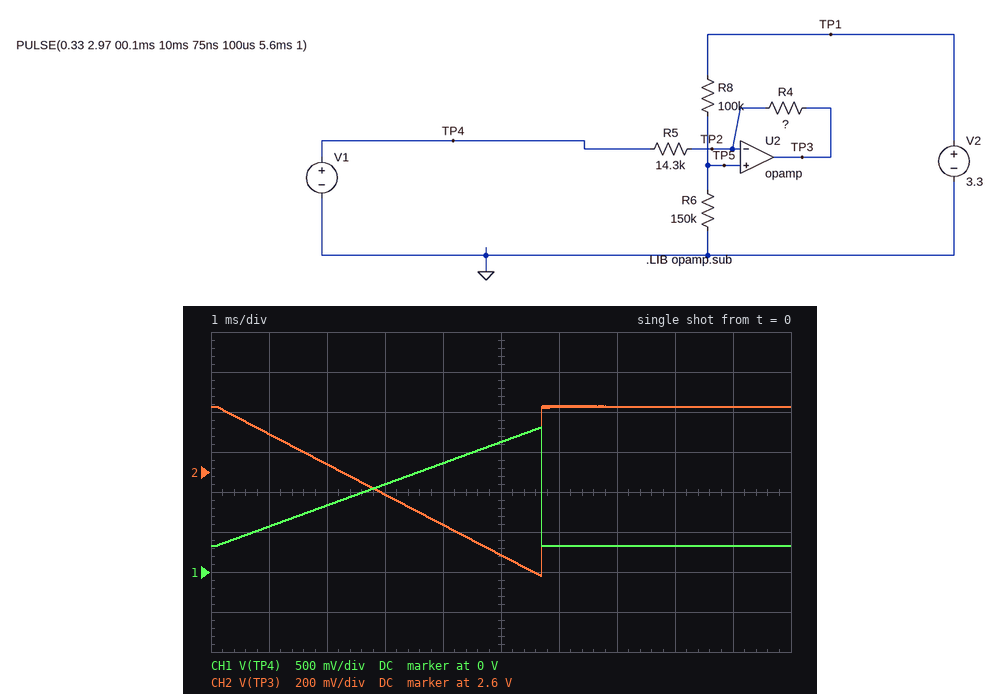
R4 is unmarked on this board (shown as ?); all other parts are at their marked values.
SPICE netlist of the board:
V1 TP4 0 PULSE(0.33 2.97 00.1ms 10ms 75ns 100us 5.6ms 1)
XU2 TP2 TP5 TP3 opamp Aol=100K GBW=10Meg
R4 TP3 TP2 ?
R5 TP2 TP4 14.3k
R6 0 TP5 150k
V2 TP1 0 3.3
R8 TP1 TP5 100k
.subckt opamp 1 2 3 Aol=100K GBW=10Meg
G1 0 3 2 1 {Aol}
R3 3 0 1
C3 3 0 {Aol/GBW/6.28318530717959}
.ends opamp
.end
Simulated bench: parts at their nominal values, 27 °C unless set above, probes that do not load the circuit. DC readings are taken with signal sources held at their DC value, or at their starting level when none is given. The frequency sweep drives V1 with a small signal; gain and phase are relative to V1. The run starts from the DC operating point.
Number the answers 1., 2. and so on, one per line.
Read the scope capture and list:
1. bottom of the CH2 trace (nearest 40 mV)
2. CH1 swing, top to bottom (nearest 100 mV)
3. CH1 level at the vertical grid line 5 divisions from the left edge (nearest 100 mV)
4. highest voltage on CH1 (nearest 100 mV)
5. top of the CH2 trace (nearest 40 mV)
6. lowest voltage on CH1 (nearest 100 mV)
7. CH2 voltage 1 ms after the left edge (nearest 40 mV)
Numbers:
1. 2.08 V
2. 1.5 V
3. 1.6 V
4. 1.8 V
5. 2.92 V
6. 300 mV
7. 2.80 V
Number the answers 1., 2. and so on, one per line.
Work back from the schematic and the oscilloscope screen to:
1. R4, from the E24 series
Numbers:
1. 8.2 kΩ
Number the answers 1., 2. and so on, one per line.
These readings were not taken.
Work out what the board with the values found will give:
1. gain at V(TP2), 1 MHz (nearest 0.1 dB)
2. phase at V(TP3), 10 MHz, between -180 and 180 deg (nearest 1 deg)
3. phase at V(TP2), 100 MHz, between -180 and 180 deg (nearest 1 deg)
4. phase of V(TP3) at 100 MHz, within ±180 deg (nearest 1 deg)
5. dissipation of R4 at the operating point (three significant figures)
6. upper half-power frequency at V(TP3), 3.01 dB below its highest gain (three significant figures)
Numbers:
1. -24.9 dB
2. 122 deg
3. 4 deg
4. 94 deg
5. 109 µW
6. 6.36 MHz
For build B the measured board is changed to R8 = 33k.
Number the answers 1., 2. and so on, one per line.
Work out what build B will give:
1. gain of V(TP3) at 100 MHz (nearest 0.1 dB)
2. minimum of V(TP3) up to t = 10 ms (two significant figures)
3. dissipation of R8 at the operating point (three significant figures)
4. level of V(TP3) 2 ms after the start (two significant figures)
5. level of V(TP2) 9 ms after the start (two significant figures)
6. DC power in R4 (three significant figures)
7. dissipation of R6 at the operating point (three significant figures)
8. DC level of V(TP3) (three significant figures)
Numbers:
1. -28.8 dB
2. 3.2 V
3. 10.7 µW
4. 3.8 V
5. 2.7 V
6. 226 µW
7. 48.8 µW
8. 4.07 V
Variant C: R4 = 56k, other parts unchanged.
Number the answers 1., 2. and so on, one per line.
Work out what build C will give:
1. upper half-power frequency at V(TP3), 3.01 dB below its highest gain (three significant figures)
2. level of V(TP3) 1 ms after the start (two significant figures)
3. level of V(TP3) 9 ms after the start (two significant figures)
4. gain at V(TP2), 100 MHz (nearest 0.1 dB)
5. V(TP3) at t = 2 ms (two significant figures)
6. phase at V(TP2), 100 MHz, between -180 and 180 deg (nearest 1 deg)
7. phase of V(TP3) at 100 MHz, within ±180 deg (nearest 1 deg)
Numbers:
1. 2.03 MHz
2. 7.5 V
3. 8.4 V
4. -2.0 dB
5. 6.5 V
6. 1 deg
7. 91 deg
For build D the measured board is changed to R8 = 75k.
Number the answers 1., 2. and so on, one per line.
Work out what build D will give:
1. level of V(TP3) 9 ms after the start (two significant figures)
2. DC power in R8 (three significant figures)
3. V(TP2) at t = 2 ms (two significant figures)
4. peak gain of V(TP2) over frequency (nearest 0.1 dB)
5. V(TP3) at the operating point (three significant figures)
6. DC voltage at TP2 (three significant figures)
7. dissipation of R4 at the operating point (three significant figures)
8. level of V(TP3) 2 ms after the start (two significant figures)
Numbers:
1. 3.3 V
2. 16.1 µW
3. 2.2 V
4. -8.8 dB
5. 3.27 V
6. 2.20 V
7. 140 µW
8. 3.0 V
